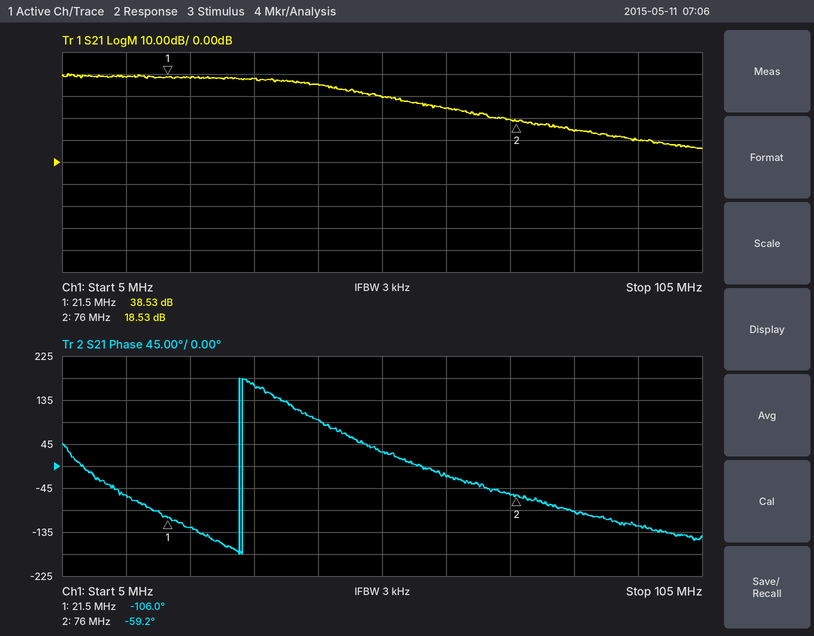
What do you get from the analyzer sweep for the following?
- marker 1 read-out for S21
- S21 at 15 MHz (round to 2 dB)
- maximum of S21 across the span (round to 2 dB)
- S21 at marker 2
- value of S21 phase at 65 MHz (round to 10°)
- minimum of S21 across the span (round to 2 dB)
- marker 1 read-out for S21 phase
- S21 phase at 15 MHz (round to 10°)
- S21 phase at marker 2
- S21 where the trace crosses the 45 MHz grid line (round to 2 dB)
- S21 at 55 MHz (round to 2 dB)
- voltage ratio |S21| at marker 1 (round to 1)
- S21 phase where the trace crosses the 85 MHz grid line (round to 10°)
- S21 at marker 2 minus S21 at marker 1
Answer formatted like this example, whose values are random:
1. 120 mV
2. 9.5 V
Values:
1. 38.53 dB
2. 38 dB
3. 40 dB
4. 18.53 dB
5. -20°
6. 6 dB
7. -106.0°
8. -60°
9. -59.2°
10. 36 dB
11. 30 dB
12. 84
13. -90°
14. -20.00 dB
